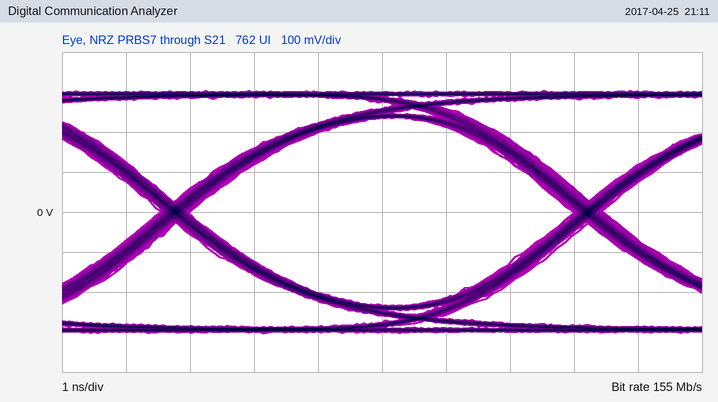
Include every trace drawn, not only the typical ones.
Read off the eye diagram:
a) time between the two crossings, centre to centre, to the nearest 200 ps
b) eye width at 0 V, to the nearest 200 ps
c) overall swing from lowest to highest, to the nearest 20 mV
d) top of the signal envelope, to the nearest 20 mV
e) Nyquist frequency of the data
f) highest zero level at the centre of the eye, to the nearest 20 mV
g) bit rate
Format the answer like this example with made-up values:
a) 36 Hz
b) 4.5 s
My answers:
a) 6.4 ns
b) 6.0 ns
c) 600 mV
d) 300 mV
e) 77.5 MHz
f) -240 mV
g) 155 Mb/s
